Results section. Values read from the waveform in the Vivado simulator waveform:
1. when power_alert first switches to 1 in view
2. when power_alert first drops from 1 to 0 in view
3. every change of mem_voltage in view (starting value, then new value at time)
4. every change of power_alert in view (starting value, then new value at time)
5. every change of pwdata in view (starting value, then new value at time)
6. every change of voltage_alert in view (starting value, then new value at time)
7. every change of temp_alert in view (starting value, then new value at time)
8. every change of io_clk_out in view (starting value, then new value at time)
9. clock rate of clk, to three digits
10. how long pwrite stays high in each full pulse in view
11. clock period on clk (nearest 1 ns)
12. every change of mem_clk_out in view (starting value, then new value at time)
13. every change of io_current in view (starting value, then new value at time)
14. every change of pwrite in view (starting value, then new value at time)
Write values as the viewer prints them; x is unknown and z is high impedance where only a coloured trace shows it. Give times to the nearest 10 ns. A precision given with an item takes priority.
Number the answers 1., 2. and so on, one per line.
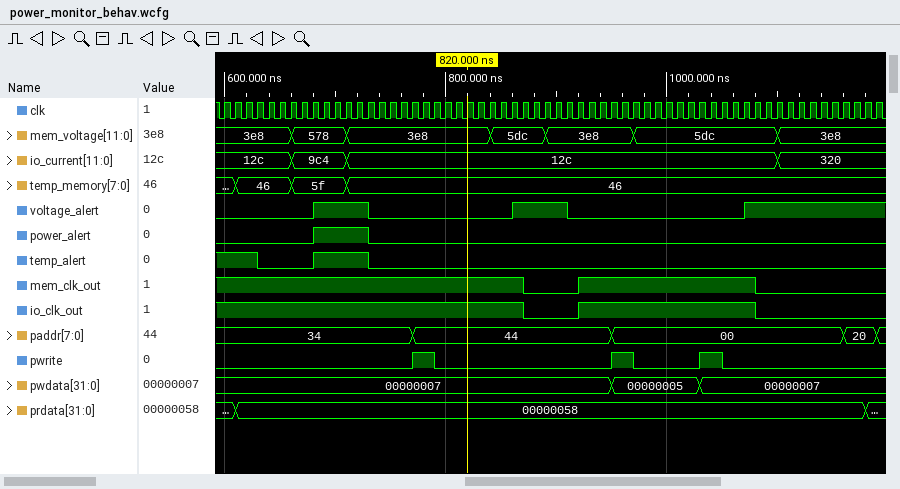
1. 680 ns
2. 730 ns
3. 3e8, 578 at 660 ns, 3e8 at 710 ns, 5dc at 840 ns, 3e8 at 890 ns, 5dc at 970 ns, 3e8 at 1100 ns
4. 0, 1 at 680 ns, 0 at 730 ns
5. 00000007, 00000005 at 950 ns, 00000007 at 1030 ns
6. 0, 1 at 680 ns, 0 at 730 ns, 1 at 860 ns, 0 at 910 ns, 1 at 1070 ns
7. 1, 0 at 630 ns, 1 at 680 ns, 0 at 730 ns
8. 1, 0 at 870 ns, 1 at 920 ns, 0 at 1080 ns
9. 100 MHz
10. 20 ns, 20 ns, 20 ns
11. 10 ns
12. 1, 0 at 870 ns, 1 at 920 ns, 0 at 1080 ns
13. 12c, 9c4 at 660 ns, 12c at 710 ns, 320 at 1100 ns
14. 0, 1 at 770 ns, 0 at 790 ns, 1 at 950 ns, 0 at 970 ns, 1 at 1030 ns, 0 at 1050 ns
